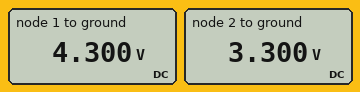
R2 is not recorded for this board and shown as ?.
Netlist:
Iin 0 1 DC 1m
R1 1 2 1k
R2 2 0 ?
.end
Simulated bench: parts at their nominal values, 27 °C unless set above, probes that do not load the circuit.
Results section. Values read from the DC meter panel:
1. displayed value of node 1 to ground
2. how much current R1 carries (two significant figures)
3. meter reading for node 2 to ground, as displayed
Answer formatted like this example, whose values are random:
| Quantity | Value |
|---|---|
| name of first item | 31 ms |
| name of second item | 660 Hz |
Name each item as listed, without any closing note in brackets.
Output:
| Quantity | Value |
|---|---|
| displayed value of node 1 to ground | 4.300 V |
| how much current R1 carries | 1.0 mA |
| meter reading for node 2 to ground, as displayed | 3.300 V |
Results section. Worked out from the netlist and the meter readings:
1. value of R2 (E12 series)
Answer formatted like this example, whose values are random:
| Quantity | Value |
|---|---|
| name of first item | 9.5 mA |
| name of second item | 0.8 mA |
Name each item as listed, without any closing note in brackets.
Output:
| Quantity | Value |
|---|---|
| value of R2 | 3.3 kΩ |
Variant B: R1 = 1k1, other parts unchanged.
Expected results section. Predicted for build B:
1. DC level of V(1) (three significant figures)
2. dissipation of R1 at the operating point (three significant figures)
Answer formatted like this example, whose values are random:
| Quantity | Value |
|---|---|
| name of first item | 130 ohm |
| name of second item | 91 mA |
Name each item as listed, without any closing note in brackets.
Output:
| Quantity | Value |
|---|---|
| DC level of V(1) | 4.40 V |
| dissipation of R1 at the operating point | 1.10 mW |
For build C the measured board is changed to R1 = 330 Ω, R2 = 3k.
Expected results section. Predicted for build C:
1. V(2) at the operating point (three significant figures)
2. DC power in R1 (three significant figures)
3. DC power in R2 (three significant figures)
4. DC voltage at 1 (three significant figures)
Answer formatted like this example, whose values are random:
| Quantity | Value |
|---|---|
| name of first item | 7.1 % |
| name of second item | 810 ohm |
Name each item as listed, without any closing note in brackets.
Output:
| Quantity | Value |
|---|---|
| V(2) at the operating point | 3.00 V |
| DC power in R1 | 330 µW |
| DC power in R2 | 3.00 mW |
| DC voltage at 1 | 3.33 V |
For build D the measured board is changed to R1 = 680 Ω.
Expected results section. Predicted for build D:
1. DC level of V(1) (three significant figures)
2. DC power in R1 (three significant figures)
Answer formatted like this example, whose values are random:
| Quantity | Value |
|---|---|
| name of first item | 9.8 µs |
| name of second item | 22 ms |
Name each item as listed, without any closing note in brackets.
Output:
| Quantity | Value |
|---|---|
| DC level of V(1) | 3.98 V |
| DC power in R1 | 680 µW |
